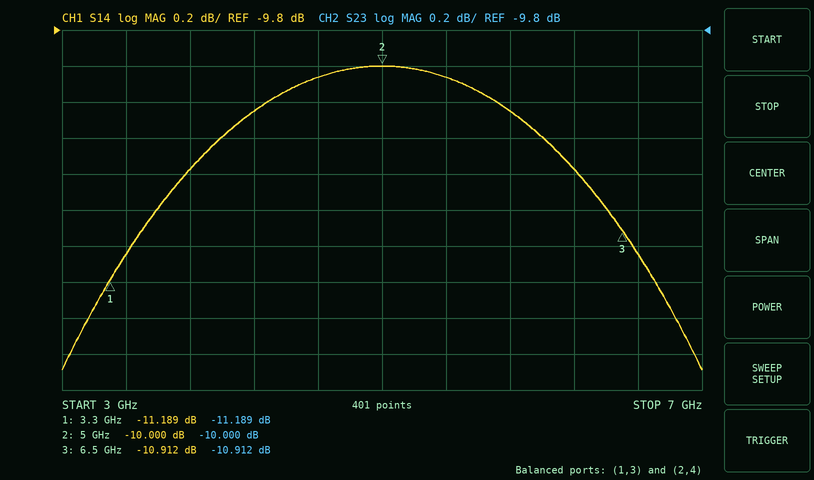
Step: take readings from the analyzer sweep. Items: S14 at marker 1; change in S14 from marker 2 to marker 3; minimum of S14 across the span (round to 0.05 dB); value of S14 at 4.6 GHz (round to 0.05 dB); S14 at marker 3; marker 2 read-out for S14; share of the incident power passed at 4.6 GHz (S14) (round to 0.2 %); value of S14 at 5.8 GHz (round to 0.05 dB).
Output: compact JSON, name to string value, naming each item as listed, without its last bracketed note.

{"S14 at marker 1": "-11.189 dB", "change in S14 from marker 2 to marker 3": "-0.912 dB", "minimum of S14 across the span": "-11.70 dB", "value of S14 at 4.6 GHz": "-10.05 dB", "S14 at marker 3": "-10.912 dB", "marker 2 read-out for S14": "-10.000 dB", "share of the incident power passed at 4.6 GHz (S14)": "9.8 %", "value of S14 at 5.8 GHz": "-10.25 dB"}
